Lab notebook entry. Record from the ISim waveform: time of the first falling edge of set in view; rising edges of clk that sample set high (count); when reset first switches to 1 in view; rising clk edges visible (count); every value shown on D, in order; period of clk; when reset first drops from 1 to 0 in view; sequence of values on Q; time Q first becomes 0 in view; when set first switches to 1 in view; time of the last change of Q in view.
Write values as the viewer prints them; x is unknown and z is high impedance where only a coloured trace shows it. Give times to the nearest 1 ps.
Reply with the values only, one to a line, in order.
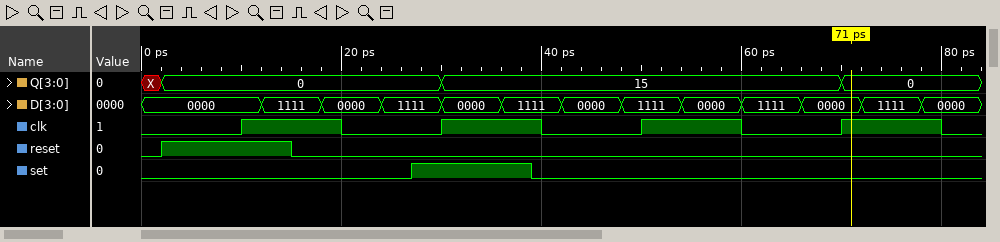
39 ps
1
2 ps
4
0000, 1111, 0000, 1111, 0000, 1111, 0000, 1111, 0000, 1111, 0000, 1111, 0000
20 ps
15 ps
X, 0, 15, 0
2 ps
27 ps
70 ps
